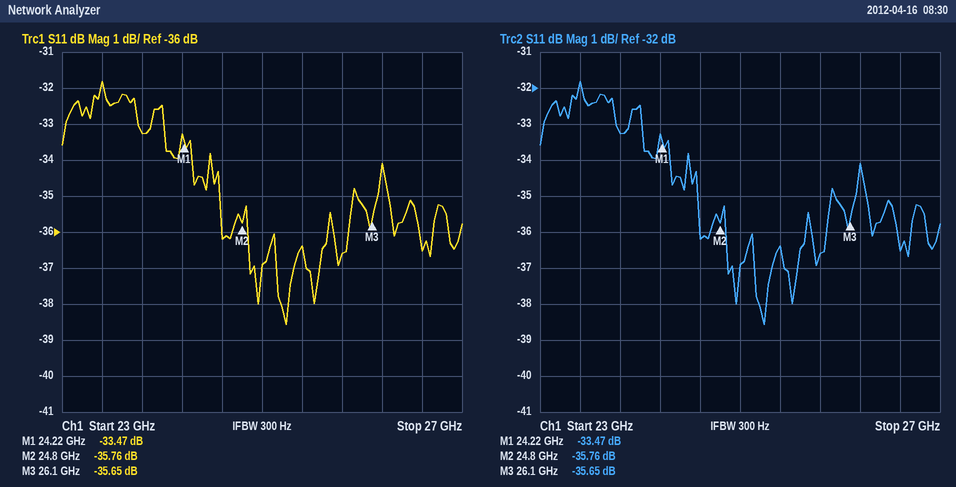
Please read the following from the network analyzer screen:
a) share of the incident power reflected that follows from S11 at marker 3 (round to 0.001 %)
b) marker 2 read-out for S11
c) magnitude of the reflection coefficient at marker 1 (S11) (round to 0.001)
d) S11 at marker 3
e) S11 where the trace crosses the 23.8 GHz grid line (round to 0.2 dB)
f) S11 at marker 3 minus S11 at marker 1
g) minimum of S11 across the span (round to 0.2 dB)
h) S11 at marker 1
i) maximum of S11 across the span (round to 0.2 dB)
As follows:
0.027 %
-35.76 dB
0.021
-35.65 dB
-33.2 dB
-2.18 dB
-38.6 dB
-33.47 dB
-31.8 dB
